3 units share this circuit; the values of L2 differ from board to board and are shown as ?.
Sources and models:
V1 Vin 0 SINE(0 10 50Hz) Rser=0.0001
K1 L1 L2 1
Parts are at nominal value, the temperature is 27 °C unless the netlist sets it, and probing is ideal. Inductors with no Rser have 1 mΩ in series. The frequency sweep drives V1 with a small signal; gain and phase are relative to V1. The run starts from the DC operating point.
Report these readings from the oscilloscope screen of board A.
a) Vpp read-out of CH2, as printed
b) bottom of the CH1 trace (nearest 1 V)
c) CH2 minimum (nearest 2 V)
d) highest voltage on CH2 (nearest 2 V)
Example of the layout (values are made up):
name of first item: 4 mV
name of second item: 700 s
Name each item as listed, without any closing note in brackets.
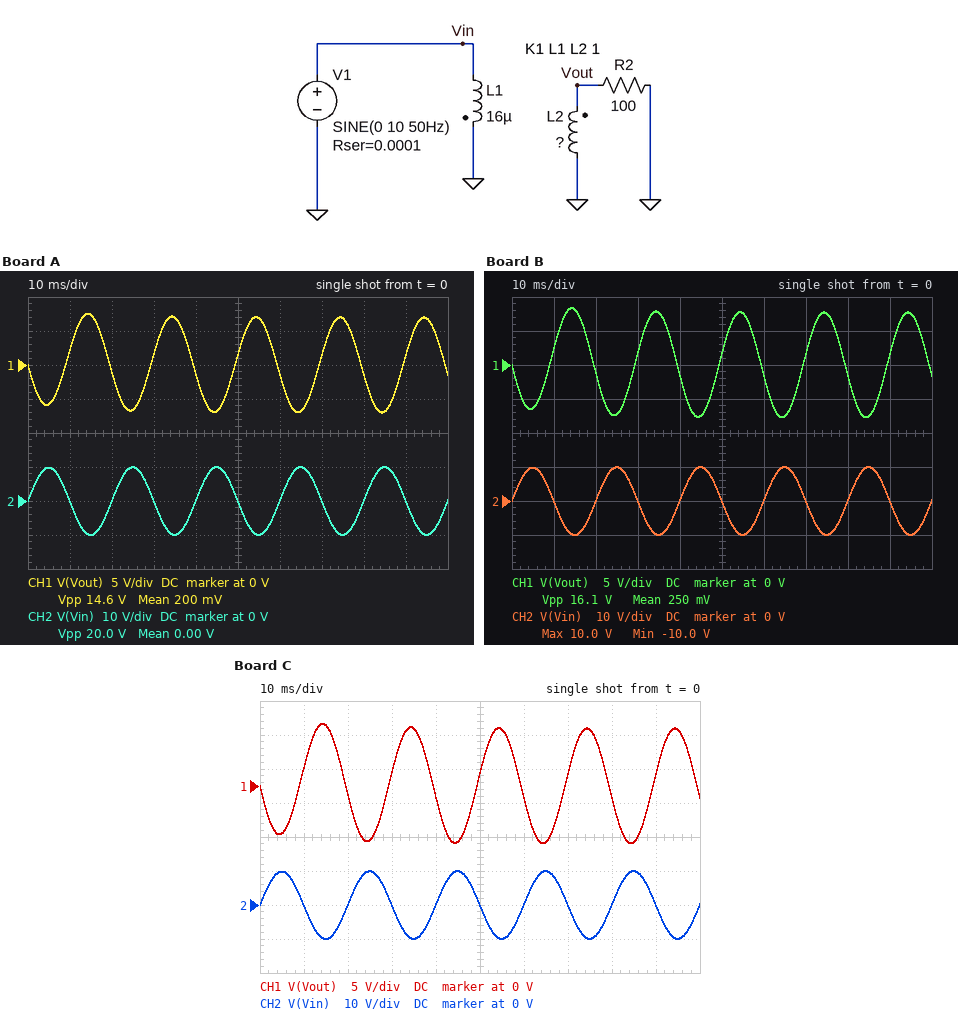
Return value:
Vpp read-out of CH2, as printed: 20.0 V
bottom of the CH1 trace: -7 V
CH2 minimum: -10 V
highest voltage on CH2: 10 V
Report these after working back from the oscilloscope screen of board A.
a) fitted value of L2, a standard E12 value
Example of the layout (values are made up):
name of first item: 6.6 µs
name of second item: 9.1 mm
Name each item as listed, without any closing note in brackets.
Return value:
fitted value of L2, a standard E12 value: 8.2 µH
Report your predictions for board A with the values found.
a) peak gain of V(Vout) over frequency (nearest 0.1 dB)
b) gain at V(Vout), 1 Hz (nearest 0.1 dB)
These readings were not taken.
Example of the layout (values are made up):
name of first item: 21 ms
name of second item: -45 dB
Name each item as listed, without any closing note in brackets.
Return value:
peak gain of V(Vout) over frequency: -2.9 dB
gain at V(Vout), 1 Hz: -23.7 dB
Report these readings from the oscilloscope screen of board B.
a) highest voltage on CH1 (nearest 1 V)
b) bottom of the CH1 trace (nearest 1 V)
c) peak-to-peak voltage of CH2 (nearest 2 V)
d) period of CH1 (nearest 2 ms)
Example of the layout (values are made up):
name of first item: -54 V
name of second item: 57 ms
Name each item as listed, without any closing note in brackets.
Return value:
highest voltage on CH1: 8 V
bottom of the CH1 trace: -8 V
peak-to-peak voltage of CH2: 20 V
period of CH1: 20 ms
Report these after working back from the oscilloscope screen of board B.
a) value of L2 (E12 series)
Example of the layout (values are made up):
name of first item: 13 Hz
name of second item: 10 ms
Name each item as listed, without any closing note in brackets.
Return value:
value of L2: 10 µH
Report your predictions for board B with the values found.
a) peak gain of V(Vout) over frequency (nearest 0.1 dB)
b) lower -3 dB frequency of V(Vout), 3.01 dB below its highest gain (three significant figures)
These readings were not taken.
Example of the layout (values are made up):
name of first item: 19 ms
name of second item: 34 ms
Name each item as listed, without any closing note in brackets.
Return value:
peak gain of V(Vout) over frequency: -2.0 dB
lower -3 dB frequency of V(Vout), 3.01 dB below its highest gain: 10.9 Hz
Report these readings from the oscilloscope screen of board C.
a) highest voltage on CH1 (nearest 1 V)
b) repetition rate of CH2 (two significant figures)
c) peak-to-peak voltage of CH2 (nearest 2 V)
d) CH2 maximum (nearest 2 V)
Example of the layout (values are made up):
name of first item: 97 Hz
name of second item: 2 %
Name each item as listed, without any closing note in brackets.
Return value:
highest voltage on CH1: 9 V
repetition rate of CH2: 50 Hz
peak-to-peak voltage of CH2: 20 V
CH2 maximum: 10 V
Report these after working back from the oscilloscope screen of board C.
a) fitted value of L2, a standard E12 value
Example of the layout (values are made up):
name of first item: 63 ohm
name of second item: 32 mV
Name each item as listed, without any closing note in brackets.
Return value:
fitted value of L2, a standard E12 value: 12 µH
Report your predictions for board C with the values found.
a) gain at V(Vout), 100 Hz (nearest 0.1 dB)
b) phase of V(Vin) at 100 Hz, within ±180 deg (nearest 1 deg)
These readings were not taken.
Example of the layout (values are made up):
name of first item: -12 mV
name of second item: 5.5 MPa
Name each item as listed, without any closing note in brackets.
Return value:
gain at V(Vout), 100 Hz: -1.3 dB
phase of V(Vin) at 100 Hz, within ±180 deg: 1 deg
